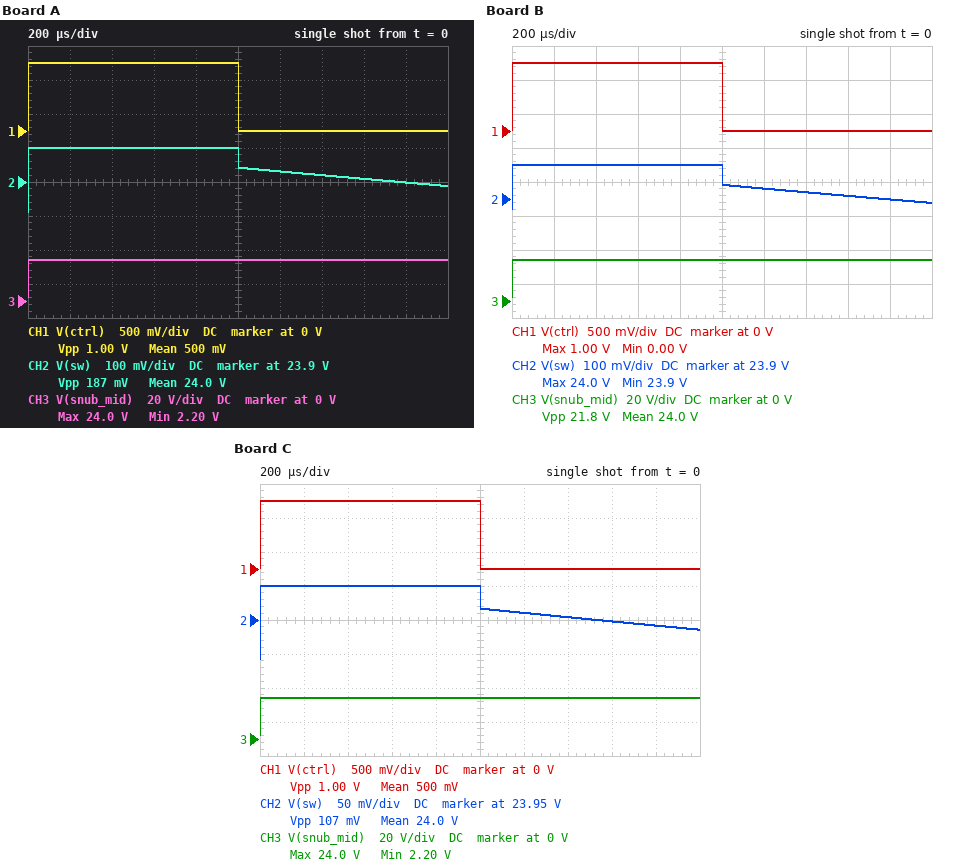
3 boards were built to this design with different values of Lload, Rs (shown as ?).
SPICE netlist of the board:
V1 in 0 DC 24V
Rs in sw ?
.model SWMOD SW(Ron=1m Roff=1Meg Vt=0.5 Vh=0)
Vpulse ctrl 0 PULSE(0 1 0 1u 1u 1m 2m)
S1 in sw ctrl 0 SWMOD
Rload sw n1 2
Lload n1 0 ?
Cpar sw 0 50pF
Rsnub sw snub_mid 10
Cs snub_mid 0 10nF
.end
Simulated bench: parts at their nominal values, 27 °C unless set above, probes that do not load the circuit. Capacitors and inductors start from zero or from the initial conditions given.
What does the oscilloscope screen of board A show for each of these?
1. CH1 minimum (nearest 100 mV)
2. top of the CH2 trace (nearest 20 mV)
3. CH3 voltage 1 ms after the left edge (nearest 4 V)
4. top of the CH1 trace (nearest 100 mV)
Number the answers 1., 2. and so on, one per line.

1. 0 V
2. 24.00 V
3. 24 V
4. 1.0 V
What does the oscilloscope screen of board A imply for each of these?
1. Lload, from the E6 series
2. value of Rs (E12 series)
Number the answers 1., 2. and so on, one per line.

1. 33 mH
2. 0.082 Ω
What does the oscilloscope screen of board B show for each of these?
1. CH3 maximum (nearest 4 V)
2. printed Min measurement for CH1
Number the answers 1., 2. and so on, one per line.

1. 24 V
2. 0.00 V
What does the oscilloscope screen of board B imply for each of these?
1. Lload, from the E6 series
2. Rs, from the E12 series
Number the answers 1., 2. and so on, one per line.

1. 22 mH
2. 0.056 Ω
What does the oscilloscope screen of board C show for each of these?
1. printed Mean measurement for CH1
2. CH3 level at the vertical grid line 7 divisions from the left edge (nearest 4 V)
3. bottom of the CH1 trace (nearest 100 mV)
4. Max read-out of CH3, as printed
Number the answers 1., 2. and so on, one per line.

1. 500 mV
2. 24 V
3. 0 V
4. 24.0 V
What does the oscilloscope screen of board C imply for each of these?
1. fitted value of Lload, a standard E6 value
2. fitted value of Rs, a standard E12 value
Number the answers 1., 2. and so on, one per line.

1. 33 mH
2. 0.047 Ω
